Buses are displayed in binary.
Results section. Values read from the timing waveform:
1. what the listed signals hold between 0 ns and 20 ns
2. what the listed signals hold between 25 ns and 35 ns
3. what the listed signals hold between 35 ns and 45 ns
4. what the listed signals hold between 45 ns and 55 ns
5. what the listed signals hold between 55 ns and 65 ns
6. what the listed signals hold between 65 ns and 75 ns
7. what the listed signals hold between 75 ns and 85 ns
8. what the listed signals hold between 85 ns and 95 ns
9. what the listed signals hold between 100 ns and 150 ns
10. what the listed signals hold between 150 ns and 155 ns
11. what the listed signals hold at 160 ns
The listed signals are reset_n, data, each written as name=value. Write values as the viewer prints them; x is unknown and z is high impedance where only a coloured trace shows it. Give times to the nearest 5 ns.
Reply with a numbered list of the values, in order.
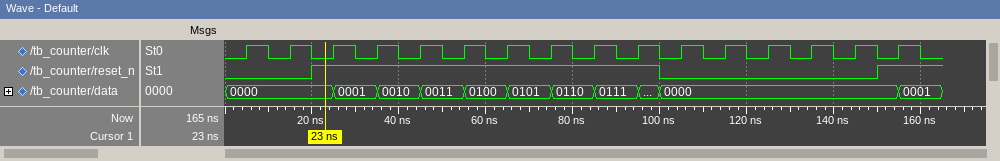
1. reset_n=0, data=0000
2. reset_n=1, data=0001
3. reset_n=1, data=0010
4. reset_n=1, data=0011
5. reset_n=1, data=0100
6. reset_n=1, data=0101
7. reset_n=1, data=0110
8. reset_n=1, data=0111
9. reset_n=0, data=0000
10. reset_n=1, data=0000
11. reset_n=1, data=0001
